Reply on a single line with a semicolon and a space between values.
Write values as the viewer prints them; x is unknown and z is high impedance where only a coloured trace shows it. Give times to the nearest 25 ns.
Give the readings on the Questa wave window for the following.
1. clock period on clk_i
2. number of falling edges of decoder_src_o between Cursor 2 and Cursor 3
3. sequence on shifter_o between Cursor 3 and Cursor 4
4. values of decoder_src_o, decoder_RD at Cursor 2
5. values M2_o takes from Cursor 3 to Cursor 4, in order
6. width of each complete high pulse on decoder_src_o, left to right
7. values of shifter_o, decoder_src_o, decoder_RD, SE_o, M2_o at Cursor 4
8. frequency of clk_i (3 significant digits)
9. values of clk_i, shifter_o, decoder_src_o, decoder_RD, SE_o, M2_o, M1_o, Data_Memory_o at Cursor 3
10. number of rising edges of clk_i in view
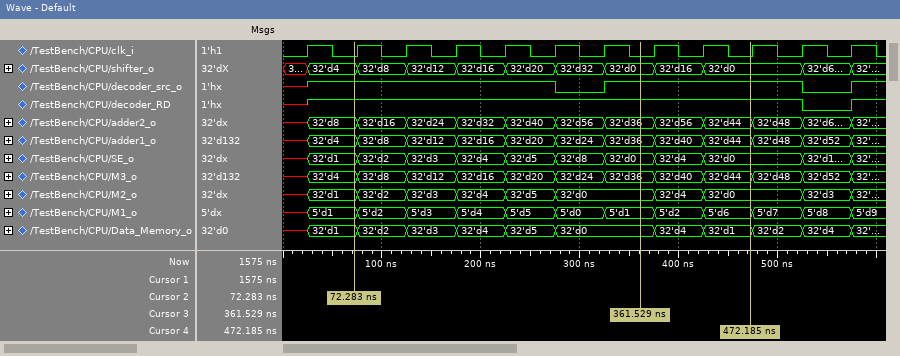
50 ns; 1; 32'd0, 32'd16, 32'd0; decoder_src_o=1, decoder_RD=1; 32'd0, 32'd4, 32'd0; 200 ns; shifter_o=32'd0, decoder_src_o=1, decoder_RD=1, SE_o=32'd0, M2_o=32'd0; 20.0 MHz; clk_i=0, shifter_o=32'd0, decoder_src_o=1, decoder_RD=1, SE_o=32'd0, M2_o=32'd0, M1_o=5'd1, Data_Memory_o=32'd0; 12
